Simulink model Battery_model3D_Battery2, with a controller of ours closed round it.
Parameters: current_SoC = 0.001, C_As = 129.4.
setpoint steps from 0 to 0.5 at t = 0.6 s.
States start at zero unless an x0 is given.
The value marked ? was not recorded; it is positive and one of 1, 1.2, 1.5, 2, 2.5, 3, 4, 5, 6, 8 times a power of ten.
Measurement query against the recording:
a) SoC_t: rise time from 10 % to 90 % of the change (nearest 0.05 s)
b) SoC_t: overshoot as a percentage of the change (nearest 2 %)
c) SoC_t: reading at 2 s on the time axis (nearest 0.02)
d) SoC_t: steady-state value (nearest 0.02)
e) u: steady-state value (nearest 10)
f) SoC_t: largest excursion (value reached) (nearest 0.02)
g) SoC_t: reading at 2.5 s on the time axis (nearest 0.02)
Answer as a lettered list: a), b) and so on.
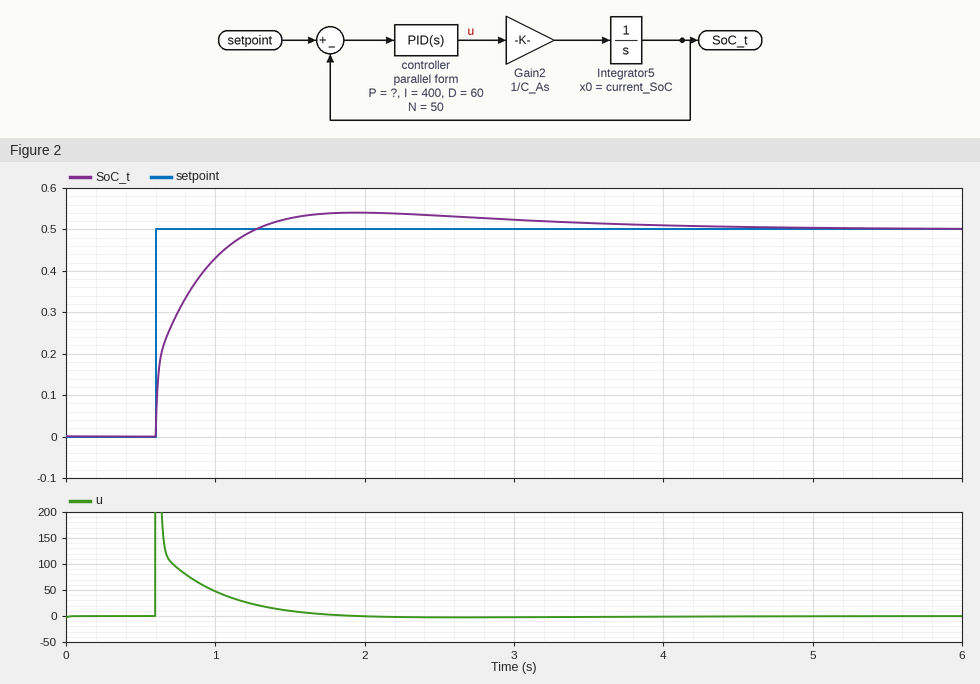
a) 0.45 s
b) 8 %
c) 0.54
d) 0.50
e) 0
f) 0.54
g) 0.54
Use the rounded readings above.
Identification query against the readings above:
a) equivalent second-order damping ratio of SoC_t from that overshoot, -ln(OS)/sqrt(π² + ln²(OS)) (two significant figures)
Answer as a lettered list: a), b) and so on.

a) 0.63
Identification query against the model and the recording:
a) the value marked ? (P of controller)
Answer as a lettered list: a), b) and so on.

a) 600
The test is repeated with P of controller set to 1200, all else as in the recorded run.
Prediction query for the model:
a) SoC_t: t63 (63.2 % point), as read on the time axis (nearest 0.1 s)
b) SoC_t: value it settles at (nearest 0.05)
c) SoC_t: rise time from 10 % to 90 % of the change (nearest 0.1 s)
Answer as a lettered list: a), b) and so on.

a) 0.7 s
b) 0.50
c) 0.3 s
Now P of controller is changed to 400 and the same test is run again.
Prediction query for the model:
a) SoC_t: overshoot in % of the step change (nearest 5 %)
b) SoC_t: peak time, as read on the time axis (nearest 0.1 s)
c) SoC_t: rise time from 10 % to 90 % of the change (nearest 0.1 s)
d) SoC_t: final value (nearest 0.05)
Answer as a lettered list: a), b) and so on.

a) 15 %
b) 2.1 s
c) 0.6 s
d) 0.50
